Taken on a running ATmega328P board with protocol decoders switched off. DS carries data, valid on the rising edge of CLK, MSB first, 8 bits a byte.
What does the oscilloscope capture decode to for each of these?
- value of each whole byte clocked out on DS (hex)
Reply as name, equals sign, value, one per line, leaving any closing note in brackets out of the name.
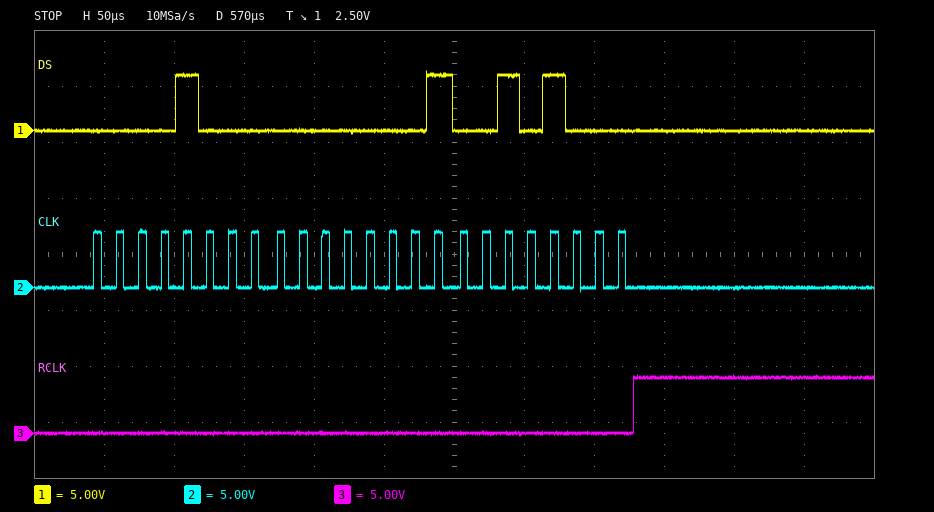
value of each whole byte clocked out on DS = 0x08 0x01 0x28
